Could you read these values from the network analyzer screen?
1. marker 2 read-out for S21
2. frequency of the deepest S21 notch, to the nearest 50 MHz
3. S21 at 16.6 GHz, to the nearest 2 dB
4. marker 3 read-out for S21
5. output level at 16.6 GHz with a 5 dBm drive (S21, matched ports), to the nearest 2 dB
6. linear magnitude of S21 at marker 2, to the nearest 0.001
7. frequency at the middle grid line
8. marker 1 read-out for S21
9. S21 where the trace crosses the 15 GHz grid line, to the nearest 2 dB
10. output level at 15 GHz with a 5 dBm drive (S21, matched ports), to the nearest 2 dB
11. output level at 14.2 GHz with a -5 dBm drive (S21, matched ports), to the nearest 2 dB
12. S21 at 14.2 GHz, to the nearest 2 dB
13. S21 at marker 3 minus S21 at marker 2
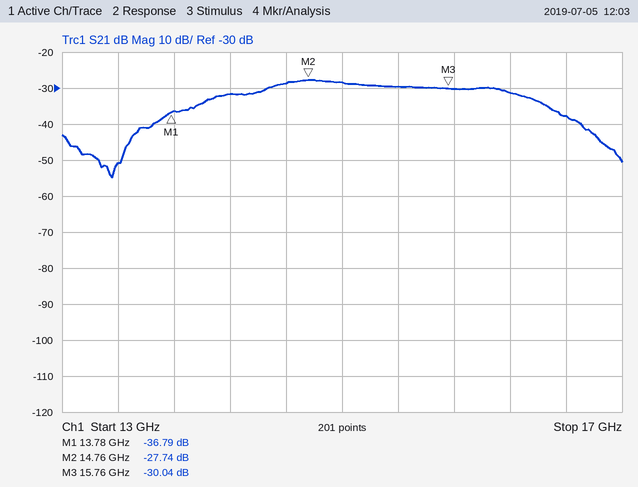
-27.74 dB
13.35 GHz
-38 dB
-30.04 dB
-32 dBm
0.041
15 GHz
-36.79 dB
-28 dB
-24 dBm
-36 dBm
-32 dB
-2.30 dB
